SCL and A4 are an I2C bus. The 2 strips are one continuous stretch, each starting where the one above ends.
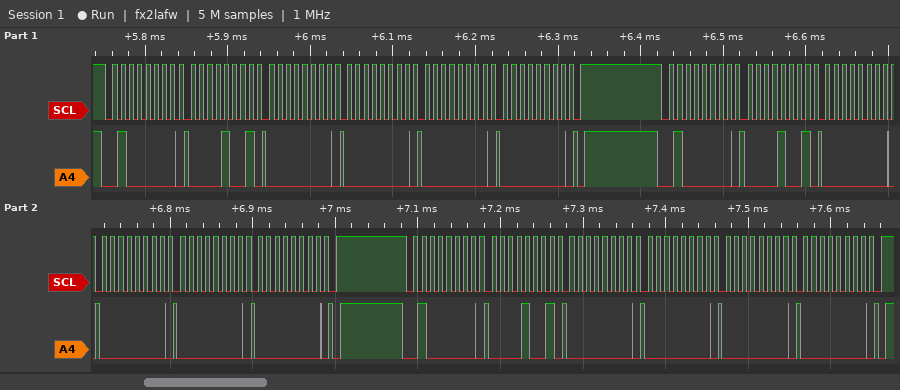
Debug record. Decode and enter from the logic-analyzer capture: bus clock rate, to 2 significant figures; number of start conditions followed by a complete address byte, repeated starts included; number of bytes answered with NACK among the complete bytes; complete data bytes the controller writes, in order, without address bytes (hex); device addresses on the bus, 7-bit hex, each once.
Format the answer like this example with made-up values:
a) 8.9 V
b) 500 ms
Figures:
a) 100 kHz
b) 3
c) 0
d) 09 00 00 00 00 09 00 00 00 00 09 00 00 00 00
e) 0x20
